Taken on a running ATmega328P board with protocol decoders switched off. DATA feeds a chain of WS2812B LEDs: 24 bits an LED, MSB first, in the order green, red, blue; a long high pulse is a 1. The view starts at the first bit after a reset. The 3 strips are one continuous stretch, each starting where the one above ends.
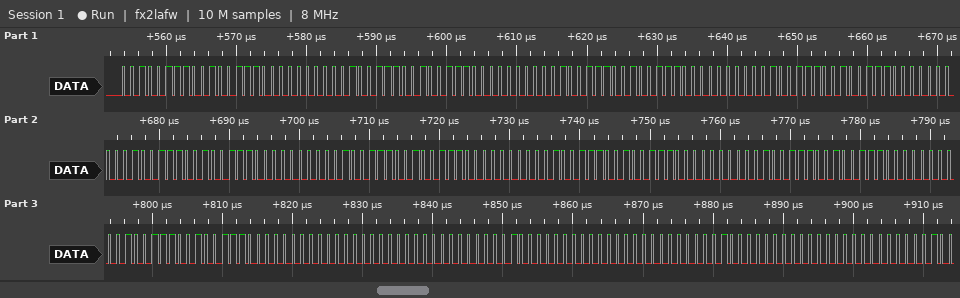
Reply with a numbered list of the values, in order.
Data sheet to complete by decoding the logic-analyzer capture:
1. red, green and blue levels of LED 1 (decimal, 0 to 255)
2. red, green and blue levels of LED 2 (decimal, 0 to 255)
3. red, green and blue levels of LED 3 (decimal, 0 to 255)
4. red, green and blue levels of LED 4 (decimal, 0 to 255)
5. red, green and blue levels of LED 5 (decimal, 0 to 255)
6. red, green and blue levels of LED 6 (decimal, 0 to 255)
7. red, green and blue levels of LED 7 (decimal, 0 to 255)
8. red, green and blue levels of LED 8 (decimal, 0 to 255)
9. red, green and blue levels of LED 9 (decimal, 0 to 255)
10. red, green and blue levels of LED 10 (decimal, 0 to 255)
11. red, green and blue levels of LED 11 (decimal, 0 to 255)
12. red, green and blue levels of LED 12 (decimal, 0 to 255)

1. 39, 39, 0
2. 39, 39, 0
3. 39, 39, 0
4. 39, 39, 0
5. 39, 39, 0
6. 39, 39, 0
7. 39, 39, 0
8. 39, 39, 0
9. 39, 39, 0
10. 0, 0, 2
11. 0, 0, 2
12. 0, 0, 2
